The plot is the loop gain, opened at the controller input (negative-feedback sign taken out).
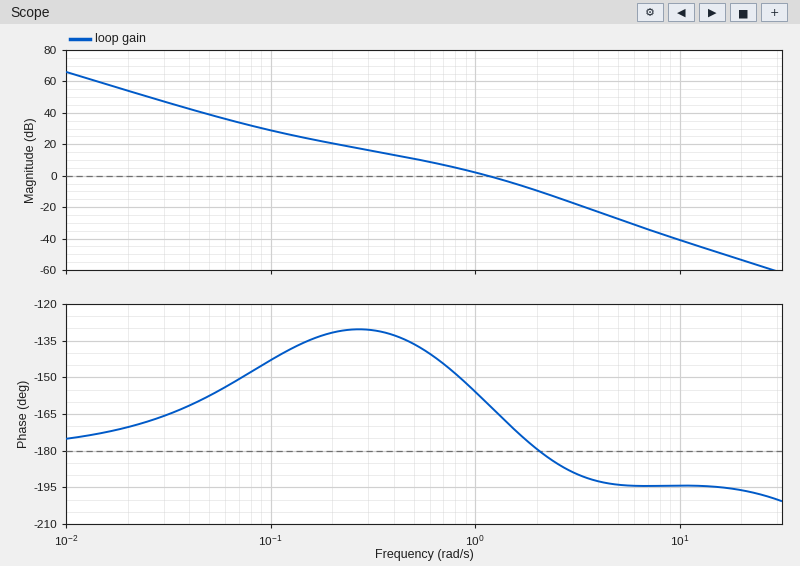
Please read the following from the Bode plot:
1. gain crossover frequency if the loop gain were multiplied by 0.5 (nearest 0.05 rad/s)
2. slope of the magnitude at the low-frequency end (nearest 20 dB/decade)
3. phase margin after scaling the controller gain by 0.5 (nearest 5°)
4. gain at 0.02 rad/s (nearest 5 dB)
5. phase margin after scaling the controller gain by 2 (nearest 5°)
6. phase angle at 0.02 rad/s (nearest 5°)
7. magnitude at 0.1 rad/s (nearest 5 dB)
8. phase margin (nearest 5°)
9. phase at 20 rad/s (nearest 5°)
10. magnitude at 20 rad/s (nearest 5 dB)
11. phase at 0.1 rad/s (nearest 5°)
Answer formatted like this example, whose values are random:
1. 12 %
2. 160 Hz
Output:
1. 0.75 rad/s
2. -40 dB/decade
3. 35°
4. 55 dB
5. 5°
6. -170°
7. 30 dB
8. 20°
9. -195°
10. -55 dB
11. -145°
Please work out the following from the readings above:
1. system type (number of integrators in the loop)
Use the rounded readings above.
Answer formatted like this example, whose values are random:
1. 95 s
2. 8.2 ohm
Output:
1. 2
